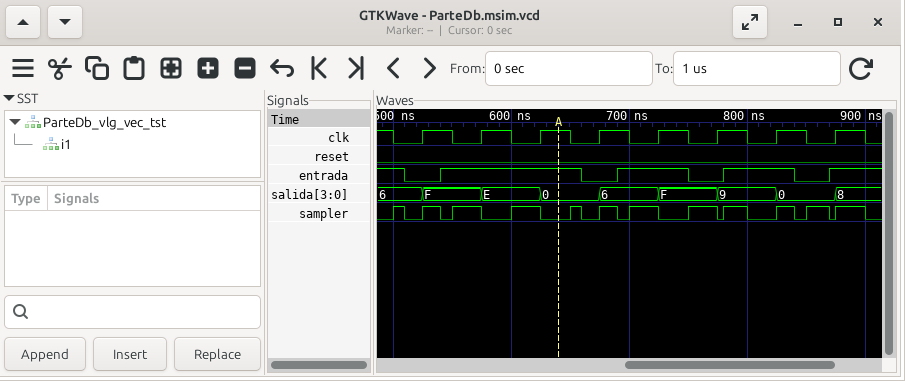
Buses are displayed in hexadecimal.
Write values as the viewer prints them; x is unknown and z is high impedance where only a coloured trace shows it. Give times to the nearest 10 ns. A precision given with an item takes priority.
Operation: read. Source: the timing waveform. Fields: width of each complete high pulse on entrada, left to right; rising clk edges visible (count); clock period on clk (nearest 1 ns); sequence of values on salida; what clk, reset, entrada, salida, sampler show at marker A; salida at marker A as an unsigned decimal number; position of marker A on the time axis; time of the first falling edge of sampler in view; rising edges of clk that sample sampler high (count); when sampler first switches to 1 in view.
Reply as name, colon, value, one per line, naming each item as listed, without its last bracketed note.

width of each complete high pulse on entrada, left to right: 120 ns, 60 ns, 60 ns
rising clk edges visible: 8
clock period on clk: 50 ns
sequence of values on salida: 6, F, E, 0, 6, F, 9, 0, 8
what clk, reset, entrada, salida, sampler show at marker A: clk=1, reset=0, entrada=1, salida=0, sampler=0
salida at marker A as an unsigned decimal number: 0
position of marker A on the time axis: 640 ns
time of the first falling edge of sampler in view: 510 ns
rising edges of clk that sample sampler high: 4
when sampler first switches to 1 in view: 500 ns
